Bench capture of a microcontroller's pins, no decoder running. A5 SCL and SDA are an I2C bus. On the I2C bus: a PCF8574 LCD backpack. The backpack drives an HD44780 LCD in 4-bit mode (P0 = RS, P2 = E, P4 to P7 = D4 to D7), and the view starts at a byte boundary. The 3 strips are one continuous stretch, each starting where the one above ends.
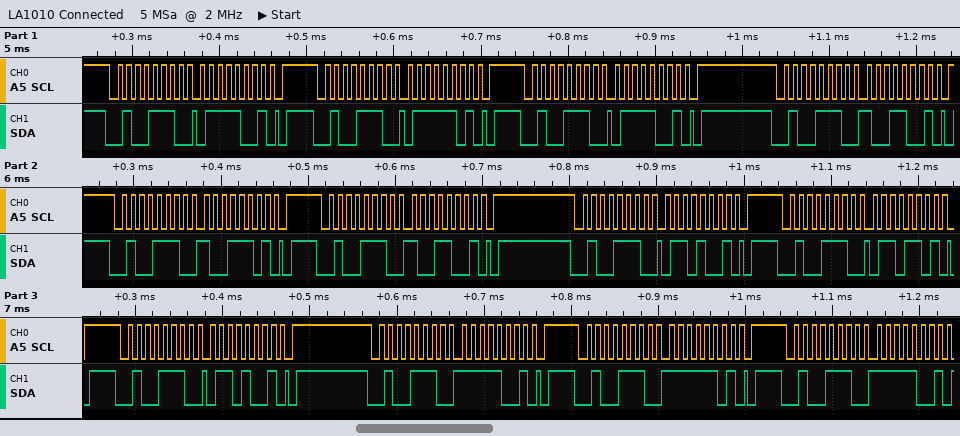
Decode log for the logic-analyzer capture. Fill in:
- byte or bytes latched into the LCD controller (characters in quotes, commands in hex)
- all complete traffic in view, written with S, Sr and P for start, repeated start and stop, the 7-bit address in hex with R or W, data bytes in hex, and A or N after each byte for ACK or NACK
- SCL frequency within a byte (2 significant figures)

'y' 'o'
S 27W A 79 A P S 27W A 7D A P S 27W A 79 A P S 27W A 99 A P S 27W A 9D A P S 27W A 99 A P S 27W A 69 A P S 27W A 6D A P S 27W A 69 A P S 27W A F9 A P S 27W A FD A P S 27W A F9 A
100 kHz
